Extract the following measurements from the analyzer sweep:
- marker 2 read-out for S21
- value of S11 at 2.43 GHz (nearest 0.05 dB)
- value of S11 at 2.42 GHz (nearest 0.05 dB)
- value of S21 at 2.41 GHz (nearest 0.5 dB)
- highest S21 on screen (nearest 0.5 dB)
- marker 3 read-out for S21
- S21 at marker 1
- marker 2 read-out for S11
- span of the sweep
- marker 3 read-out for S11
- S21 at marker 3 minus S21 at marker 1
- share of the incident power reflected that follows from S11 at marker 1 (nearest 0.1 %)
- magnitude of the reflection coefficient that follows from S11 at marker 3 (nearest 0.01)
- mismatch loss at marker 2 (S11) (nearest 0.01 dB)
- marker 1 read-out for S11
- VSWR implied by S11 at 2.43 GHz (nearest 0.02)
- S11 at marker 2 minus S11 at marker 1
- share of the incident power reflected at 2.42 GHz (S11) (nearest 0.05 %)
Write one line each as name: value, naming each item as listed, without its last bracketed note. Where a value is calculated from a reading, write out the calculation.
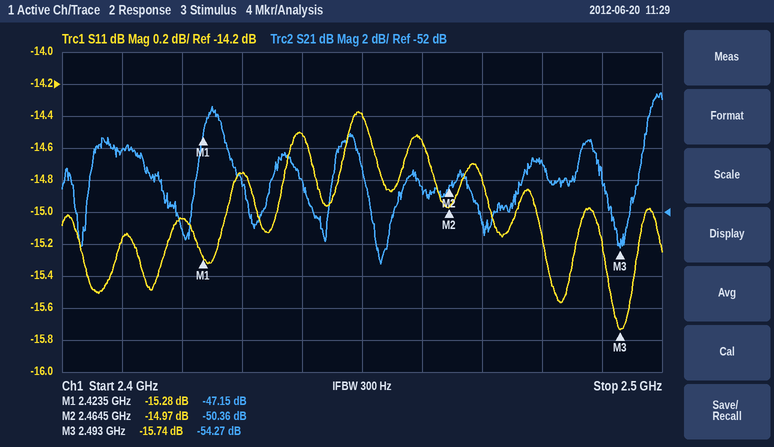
marker 2 read-out for S21: -50.36 dB
value of S11 at 2.43 GHz: -14.75 dB
value of S11 at 2.42 GHz: -15.05 dB
value of S21 at 2.41 GHz: -48.0 dB
highest S21 on screen: -44.5 dB
marker 3 read-out for S21: -54.27 dB
S21 at marker 1: -47.15 dB
marker 2 read-out for S11: -14.97 dB
span of the sweep: 100 MHz
marker 3 read-out for S11: -15.74 dB
S21 at marker 3 minus S21 at marker 1: -54.27 − (-47.15) = -7.12 dB
share of the incident power reflected that follows from S11 at marker 1: 10^(-15.28/10) ≈ 3.0 %
magnitude of the reflection coefficient that follows from S11 at marker 3: 10^(-15.74/20) ≈ 0.16
mismatch loss at marker 2 (S11): −10 log10(1 − 10^(-14.97/10)) ≈ 0.14 dB
marker 1 read-out for S11: -15.28 dB
VSWR implied by S11 at 2.43 GHz: |Γ| = 10^(-14.75/20) = 0.1830; VSWR = (1 + 0.1830)/(1 − 0.1830) ≈ 1.45, so 1.44 to the nearest 0.02
S11 at marker 2 minus S11 at marker 1: -14.97 − (-15.28) = 0.31 dB
share of the incident power reflected at 2.42 GHz (S11): 10^(-15.05/10) ≈ 3.13 %, so 3.15 % to the nearest 0.05 %
